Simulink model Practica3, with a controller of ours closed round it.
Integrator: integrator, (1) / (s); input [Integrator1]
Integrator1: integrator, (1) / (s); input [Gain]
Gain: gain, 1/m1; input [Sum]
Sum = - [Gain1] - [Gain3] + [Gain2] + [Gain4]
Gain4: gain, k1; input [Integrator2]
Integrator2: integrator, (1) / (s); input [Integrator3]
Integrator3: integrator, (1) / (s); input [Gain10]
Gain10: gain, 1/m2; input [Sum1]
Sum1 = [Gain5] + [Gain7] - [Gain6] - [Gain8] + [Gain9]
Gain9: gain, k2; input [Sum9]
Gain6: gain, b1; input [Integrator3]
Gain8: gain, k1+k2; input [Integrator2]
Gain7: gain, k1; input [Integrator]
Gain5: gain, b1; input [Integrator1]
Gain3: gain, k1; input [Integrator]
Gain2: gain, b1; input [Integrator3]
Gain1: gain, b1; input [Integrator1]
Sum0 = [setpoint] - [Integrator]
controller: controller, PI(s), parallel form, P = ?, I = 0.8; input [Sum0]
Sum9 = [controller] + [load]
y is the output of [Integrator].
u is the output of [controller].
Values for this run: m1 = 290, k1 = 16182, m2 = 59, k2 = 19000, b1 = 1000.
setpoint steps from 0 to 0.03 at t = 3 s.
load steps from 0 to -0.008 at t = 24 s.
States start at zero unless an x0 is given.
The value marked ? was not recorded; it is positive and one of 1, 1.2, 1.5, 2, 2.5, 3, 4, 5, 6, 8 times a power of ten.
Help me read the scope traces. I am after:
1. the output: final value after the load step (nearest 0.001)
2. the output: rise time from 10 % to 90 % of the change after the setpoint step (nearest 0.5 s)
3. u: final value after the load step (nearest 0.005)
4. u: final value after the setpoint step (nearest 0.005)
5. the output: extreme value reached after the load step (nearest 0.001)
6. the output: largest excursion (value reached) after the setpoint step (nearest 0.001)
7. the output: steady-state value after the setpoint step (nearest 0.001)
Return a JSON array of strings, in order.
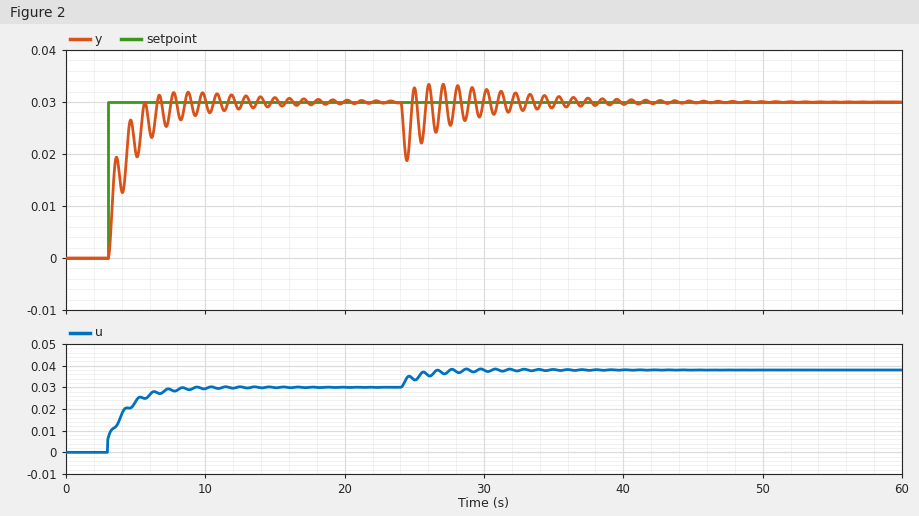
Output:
["0.030", "2.5 s", "0.040", "0.030", "0.019", "0.032", "0.030"]
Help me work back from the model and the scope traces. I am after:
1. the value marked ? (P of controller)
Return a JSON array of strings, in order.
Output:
["0.2"]
